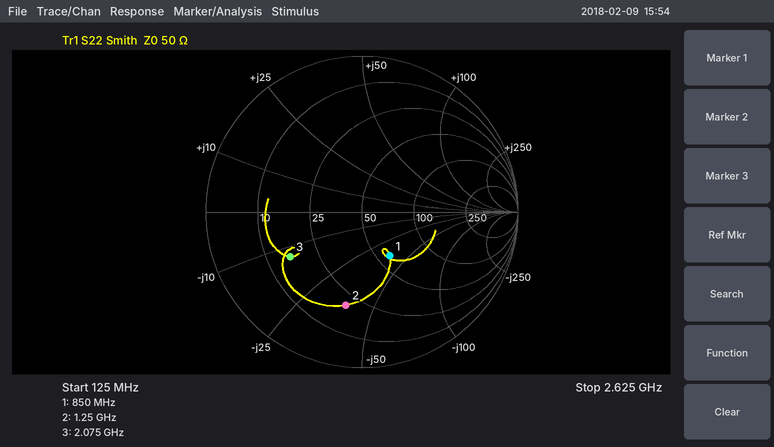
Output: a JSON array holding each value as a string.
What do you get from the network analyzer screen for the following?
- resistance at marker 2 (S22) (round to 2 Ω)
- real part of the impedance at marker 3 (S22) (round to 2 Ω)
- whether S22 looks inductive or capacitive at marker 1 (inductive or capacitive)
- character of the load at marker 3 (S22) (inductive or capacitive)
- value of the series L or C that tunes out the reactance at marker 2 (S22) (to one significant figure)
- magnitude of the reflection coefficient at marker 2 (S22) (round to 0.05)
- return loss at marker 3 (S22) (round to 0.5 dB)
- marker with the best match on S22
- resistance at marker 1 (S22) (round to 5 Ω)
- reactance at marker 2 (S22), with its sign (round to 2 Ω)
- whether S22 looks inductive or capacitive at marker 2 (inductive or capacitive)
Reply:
["20 Ω", "16 Ω", "capacitive", "capacitive", "5 nH", "0.60", "5.5 dB", "marker 1", "60 Ω", "-38 Ω", "capacitive"]
